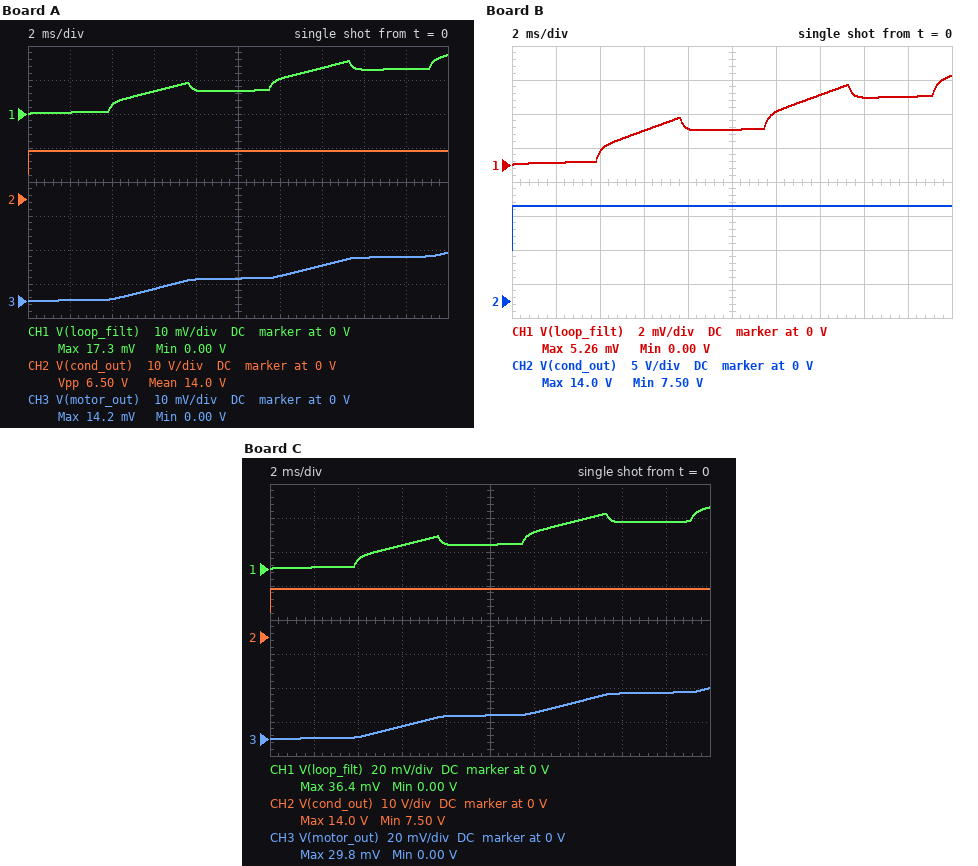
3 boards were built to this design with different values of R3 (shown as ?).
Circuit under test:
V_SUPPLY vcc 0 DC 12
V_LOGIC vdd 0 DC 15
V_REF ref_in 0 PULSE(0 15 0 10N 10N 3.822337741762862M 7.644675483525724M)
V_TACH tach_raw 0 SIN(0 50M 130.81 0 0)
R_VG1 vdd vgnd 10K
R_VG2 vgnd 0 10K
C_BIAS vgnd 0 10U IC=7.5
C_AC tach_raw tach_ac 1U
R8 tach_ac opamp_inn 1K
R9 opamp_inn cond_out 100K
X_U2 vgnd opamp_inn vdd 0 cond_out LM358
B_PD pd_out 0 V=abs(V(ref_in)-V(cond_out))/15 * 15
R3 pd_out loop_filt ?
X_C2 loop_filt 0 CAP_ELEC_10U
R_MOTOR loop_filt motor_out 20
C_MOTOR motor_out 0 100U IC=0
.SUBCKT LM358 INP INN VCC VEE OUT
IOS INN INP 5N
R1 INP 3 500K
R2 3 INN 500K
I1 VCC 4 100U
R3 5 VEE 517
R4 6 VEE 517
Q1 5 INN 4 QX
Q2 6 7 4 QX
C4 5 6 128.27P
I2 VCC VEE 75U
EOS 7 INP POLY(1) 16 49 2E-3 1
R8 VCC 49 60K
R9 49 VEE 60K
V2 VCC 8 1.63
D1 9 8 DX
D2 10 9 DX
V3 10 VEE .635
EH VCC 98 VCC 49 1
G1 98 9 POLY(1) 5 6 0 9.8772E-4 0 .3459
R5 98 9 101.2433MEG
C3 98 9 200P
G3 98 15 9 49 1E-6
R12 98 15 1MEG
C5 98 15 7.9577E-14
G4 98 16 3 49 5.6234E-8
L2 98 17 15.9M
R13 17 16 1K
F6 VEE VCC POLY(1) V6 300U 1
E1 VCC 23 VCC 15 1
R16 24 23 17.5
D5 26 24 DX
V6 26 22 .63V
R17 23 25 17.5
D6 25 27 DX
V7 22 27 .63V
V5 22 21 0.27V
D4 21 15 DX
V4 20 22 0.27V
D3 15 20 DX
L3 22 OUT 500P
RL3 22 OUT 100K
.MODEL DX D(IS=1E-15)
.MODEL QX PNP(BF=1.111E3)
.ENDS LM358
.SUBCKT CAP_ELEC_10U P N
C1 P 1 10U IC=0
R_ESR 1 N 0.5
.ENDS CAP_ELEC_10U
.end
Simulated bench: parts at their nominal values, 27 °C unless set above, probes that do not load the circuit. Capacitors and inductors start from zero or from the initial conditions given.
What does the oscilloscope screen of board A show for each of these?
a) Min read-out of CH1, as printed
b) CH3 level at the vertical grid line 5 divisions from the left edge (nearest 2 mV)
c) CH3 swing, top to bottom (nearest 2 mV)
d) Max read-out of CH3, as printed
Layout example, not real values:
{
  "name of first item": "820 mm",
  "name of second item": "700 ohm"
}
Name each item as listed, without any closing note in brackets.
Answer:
{
  "Min read-out of CH1, as printed": "0.00 V",
  "CH3 level at the vertical grid line 5 divisions from the left edge": "6 mV",
  "CH3 swing, top to bottom": "14 mV",
  "Max read-out of CH3, as printed": "14.2 mV"
}
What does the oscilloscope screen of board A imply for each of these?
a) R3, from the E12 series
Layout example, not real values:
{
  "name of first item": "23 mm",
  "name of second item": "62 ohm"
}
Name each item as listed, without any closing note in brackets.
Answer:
{
  "R3, from the E12 series": "82 kΩ"
}
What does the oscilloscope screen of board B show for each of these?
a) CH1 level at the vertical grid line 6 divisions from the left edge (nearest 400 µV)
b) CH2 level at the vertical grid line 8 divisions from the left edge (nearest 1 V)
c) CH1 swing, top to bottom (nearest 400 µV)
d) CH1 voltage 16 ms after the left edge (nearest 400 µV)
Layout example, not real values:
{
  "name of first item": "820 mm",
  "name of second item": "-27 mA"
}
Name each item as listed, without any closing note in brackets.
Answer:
{
  "CH1 level at the vertical grid line 6 divisions from the left edge": "3.2 mV",
  "CH2 level at the vertical grid line 8 divisions from the left edge": "14 V",
  "CH1 swing, top to bottom": "5.2 mV",
  "CH1 voltage 16 ms after the left edge": "4.0 mV"
}
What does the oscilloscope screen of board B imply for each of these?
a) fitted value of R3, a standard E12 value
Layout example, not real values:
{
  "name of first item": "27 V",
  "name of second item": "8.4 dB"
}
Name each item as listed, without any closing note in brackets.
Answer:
{
  "fitted value of R3, a standard E12 value": "270 kΩ"
}
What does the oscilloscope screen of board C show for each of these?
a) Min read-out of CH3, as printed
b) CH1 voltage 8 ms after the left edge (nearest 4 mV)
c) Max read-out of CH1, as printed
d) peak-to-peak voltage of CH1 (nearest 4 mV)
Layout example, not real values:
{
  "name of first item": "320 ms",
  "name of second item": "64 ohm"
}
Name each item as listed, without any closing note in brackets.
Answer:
{
  "Min read-out of CH3, as printed": "0.00 V",
  "CH1 voltage 8 ms after the left edge": "16 mV",
  "Max read-out of CH1, as printed": "36.4 mV",
  "peak-to-peak voltage of CH1": "36 mV"
}
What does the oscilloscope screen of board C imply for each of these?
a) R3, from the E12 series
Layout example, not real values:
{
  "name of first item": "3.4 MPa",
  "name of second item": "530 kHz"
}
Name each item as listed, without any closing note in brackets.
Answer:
{
  "R3, from the E12 series": "39 kΩ"
}
